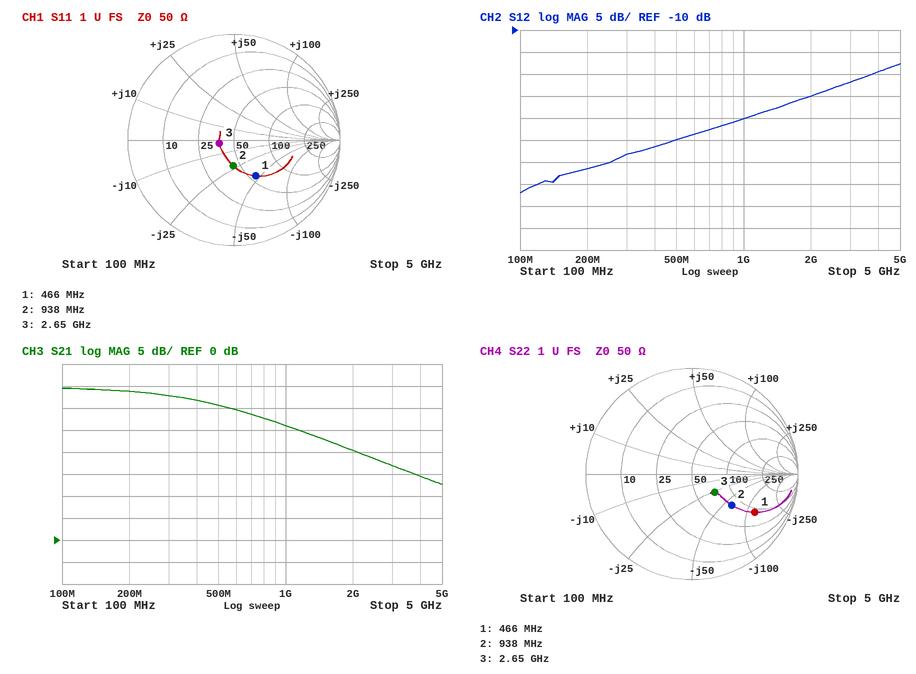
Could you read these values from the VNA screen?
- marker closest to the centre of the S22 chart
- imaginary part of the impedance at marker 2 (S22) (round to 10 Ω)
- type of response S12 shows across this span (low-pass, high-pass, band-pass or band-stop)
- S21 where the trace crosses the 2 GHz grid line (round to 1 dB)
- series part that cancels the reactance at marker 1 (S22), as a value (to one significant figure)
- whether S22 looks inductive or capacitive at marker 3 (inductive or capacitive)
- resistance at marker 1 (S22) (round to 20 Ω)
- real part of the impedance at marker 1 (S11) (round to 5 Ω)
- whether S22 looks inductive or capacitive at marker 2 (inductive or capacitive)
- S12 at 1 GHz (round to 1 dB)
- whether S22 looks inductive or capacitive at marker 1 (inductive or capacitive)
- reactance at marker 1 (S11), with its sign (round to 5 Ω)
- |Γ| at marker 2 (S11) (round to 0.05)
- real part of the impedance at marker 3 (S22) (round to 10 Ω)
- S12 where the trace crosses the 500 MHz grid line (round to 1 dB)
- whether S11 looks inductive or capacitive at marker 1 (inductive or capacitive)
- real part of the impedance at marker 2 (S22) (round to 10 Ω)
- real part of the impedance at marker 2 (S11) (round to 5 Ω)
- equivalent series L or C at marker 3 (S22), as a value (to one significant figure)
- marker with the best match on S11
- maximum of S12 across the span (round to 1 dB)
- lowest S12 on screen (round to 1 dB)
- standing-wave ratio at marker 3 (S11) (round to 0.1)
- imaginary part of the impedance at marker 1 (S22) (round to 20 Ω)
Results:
marker 3
-60 Ω
high-pass
20 dB
40 nH
capacitive
80 Ω
55 Ω
capacitive
-30 dB
capacitive
-45 Ω
0.25
70 Ω
-35 dB
capacitive
80 Ω
45 Ω
2 pF
marker 3
-18 dB
-47 dB
1.3
-120 Ω
